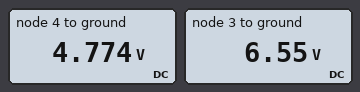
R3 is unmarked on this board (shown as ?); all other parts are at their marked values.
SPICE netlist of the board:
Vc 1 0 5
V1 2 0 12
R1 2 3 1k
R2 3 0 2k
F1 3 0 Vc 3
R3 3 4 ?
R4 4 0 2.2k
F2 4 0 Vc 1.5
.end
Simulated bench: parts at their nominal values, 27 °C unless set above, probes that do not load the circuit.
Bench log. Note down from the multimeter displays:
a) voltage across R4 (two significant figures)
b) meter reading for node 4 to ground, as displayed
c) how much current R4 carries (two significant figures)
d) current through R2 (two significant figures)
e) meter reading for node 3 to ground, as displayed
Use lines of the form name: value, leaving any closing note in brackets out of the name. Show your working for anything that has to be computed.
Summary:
voltage across R4: 4.774 V = 4.8 V
meter reading for node 4 to ground, as displayed: 4.774 V
how much current R4 carries: (4.774 V) / 2.2 kΩ = 2.2 mA
current through R2: (6.55 V) / 2 kΩ = 3.3 mA
meter reading for node 3 to ground, as displayed: 6.55 V
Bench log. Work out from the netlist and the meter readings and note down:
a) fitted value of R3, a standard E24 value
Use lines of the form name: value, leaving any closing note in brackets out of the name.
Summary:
fitted value of R3, a standard E24 value: 820 Ω
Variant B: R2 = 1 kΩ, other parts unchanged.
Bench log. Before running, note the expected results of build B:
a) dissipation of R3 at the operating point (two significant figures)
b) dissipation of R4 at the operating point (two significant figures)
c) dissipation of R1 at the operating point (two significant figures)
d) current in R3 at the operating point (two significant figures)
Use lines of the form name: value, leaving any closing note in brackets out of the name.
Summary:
dissipation of R3 at the operating point: 2.4 mW
dissipation of R4 at the operating point: 6.4 mW
dissipation of R1 at the operating point: 47 mW
current in R3 at the operating point: 1.7 mA
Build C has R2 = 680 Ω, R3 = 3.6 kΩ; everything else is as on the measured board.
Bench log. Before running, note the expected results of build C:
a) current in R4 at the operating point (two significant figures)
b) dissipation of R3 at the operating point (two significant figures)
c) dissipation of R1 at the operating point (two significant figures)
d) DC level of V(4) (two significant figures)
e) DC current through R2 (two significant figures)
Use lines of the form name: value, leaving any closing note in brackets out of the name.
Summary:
current in R4 at the operating point: 780 µA
dissipation of R3 at the operating point: 2.2 mW
dissipation of R1 at the operating point: 56 mW
DC level of V(4): 1.7 V
DC current through R2: 6.7 mA
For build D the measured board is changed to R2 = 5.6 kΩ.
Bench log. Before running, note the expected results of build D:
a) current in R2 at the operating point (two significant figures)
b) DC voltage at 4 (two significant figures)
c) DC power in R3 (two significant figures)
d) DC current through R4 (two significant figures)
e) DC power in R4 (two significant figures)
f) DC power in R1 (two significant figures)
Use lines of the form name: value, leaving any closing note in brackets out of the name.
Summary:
current in R2 at the operating point: 1.4 mA
DC voltage at 4: 5.8 V
DC power in R3: 5.7 mW
DC current through R4: 2.6 mA
DC power in R4: 15 mW
DC power in R1: 16 mW
